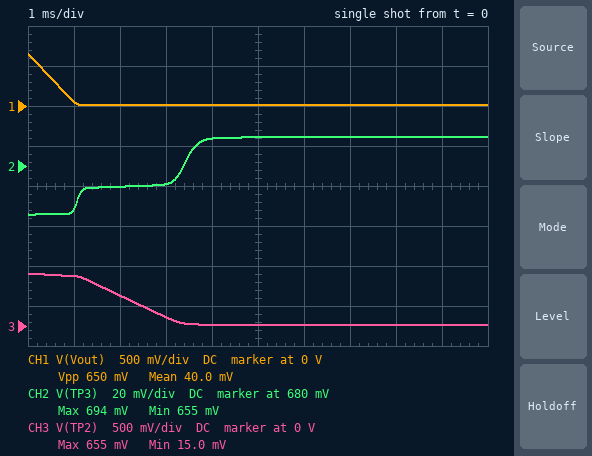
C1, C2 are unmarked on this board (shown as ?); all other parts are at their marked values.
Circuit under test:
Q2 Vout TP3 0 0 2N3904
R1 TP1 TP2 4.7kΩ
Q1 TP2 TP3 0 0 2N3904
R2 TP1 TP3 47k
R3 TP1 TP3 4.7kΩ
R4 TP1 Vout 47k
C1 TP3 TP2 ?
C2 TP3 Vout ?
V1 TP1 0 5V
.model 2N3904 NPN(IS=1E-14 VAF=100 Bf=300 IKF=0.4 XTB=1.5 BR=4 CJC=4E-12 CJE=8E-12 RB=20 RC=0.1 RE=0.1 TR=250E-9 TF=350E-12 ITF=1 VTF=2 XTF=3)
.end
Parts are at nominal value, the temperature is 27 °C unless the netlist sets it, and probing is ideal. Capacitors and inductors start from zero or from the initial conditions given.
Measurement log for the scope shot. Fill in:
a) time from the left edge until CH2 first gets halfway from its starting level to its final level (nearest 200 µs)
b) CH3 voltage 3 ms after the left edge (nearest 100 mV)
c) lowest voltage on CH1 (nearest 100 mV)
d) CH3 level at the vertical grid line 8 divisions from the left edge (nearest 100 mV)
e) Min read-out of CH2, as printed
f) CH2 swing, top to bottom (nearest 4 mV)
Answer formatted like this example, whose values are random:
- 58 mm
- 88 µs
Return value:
- 3.2 ms
- 100 mV
- 0 V
- 0 V
- 655 mV
- 40 mV
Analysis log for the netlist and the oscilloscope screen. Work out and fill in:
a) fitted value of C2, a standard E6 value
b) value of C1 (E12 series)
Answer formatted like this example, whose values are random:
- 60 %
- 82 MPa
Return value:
- 1.5 µF
- 2.7 µF
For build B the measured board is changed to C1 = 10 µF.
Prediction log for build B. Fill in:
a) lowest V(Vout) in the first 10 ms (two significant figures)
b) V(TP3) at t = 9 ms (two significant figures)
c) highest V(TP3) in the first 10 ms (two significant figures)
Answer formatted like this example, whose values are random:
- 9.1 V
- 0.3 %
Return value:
- 7.6 mV
- 670 mV
- 680 mV
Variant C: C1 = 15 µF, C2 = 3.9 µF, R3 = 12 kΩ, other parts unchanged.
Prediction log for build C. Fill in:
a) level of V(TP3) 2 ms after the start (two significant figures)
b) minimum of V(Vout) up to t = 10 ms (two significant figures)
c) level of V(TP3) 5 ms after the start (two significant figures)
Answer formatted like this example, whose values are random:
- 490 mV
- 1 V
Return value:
- 650 mV
- 8.7 mV
- 660 mV
